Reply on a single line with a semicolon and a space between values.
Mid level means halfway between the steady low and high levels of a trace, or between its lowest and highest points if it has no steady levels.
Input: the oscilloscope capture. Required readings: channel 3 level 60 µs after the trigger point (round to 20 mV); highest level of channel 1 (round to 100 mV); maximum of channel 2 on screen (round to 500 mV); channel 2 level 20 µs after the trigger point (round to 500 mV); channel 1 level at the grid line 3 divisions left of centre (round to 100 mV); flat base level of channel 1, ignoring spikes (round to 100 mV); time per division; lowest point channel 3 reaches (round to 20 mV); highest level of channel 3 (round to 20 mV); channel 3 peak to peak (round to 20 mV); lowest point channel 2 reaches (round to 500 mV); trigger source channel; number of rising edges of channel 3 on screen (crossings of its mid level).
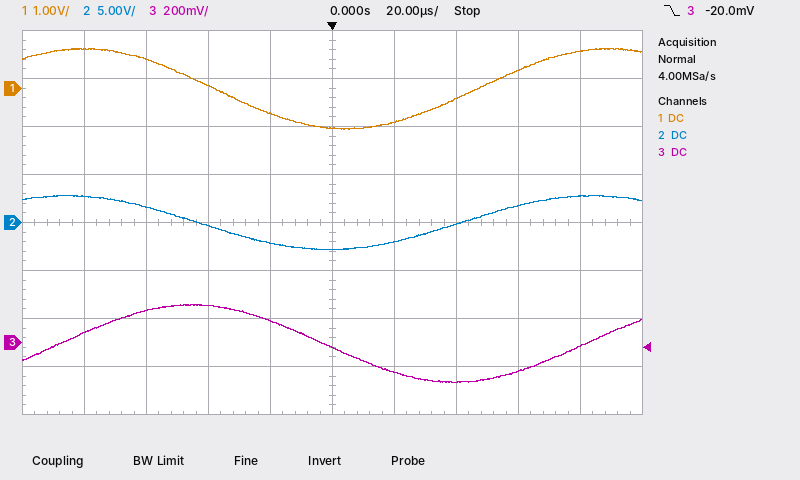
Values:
-120 mV; 800 mV; 3.0 V; -2.0 V; 600 mV; -800 mV; 20 µs; -160 mV; 160 mV; 320 mV; -3.0 V; channel 3; 2
